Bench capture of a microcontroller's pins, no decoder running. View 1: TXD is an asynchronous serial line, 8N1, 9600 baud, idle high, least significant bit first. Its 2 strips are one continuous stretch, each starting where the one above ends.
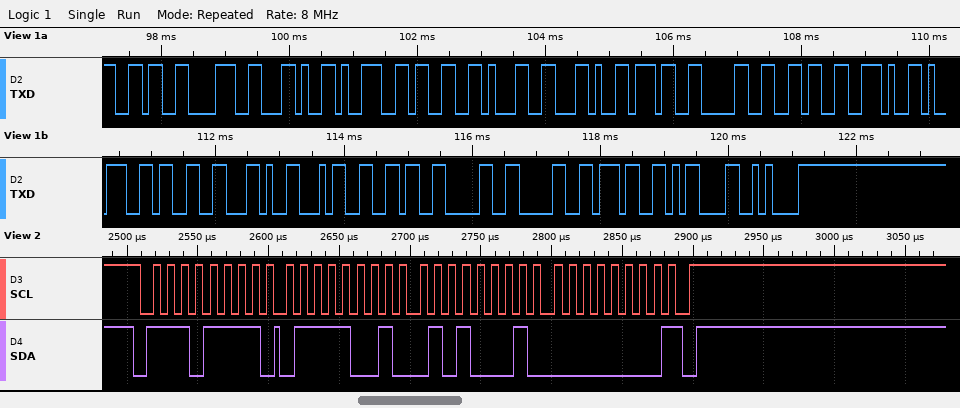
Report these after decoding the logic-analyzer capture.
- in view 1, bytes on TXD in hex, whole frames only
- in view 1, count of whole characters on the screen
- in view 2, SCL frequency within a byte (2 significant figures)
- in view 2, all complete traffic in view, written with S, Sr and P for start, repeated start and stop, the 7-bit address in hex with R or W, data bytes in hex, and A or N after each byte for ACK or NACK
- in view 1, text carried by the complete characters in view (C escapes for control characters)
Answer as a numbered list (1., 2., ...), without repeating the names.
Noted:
1. 0x36 0x38 0x2C 0x39 0x33 0x31 0x2C 0x37 0x30 0x36 0x2E 0x39 0x33 0x2C 0x34 0x36 0x30 0x30 0x37 0x0D 0x0A
2. 21
3. 100 kHz
4. S 77R A 79 A 51 A 00 N P
5. "68,931,706.93,46007\r\n"
